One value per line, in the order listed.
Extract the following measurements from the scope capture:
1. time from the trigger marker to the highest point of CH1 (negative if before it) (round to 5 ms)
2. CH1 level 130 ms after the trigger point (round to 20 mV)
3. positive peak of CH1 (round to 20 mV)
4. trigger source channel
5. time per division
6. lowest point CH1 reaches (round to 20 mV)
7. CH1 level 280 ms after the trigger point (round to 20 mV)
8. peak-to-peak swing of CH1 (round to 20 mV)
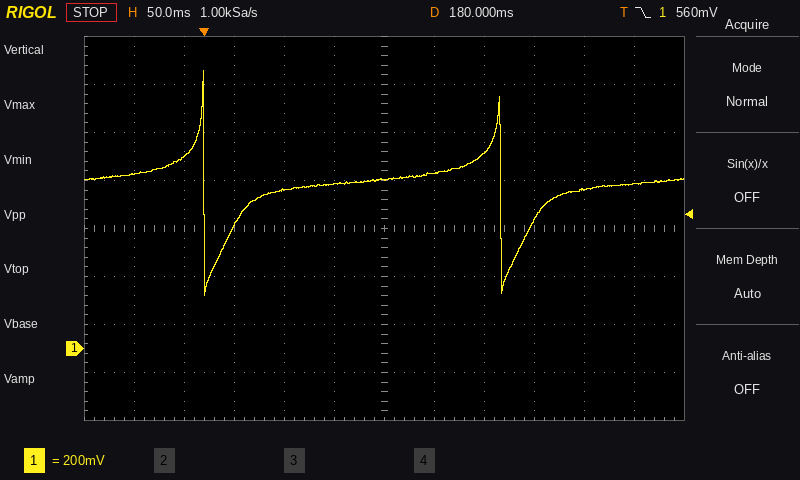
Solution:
0 ms
680 mV
1.16 V
CH1
50 ms
220 mV
820 mV
940 mV
